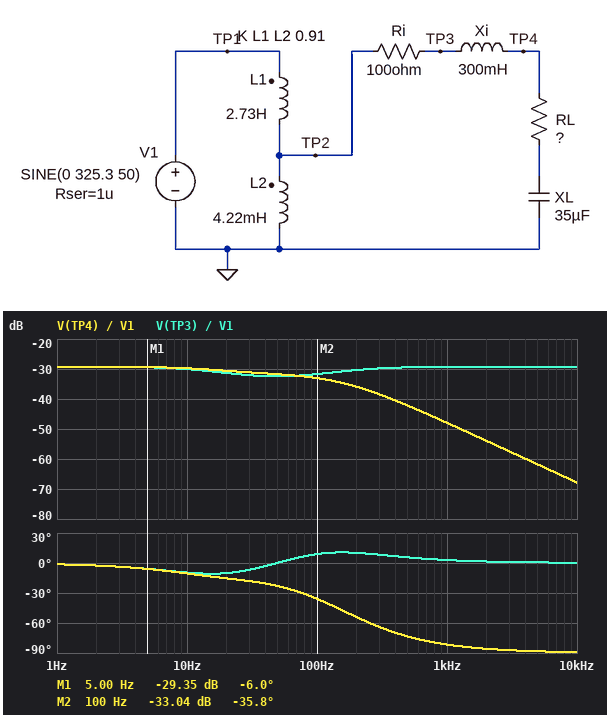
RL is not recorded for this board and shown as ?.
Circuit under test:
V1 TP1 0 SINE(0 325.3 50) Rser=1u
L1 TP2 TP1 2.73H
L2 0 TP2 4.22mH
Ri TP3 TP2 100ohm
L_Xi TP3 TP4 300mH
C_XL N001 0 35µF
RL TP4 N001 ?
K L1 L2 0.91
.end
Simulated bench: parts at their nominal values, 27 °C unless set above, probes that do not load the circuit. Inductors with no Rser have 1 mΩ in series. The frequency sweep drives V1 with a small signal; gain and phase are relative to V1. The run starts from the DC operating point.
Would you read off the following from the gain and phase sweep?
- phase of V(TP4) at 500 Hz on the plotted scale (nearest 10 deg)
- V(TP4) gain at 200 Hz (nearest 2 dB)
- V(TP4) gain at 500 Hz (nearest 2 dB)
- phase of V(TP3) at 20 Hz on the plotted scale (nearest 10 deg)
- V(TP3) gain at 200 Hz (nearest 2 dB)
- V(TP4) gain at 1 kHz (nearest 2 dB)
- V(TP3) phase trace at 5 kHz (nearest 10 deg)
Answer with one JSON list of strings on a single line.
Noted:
["-70 deg", "-36 dB", "-42 dB", "-10 deg", "-30 dB", "-48 dB", "0 deg"]
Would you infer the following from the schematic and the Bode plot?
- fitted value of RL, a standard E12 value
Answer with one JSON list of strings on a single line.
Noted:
["220 Ω"]
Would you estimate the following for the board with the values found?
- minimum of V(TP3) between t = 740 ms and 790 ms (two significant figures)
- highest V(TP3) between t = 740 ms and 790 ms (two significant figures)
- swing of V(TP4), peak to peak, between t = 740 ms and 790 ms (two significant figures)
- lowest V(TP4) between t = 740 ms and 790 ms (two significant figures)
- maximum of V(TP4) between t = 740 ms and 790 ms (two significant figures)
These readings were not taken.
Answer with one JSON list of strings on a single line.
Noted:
["-7.8 V", "7.8 V", "17 V", "-8.4 V", "8.4 V"]
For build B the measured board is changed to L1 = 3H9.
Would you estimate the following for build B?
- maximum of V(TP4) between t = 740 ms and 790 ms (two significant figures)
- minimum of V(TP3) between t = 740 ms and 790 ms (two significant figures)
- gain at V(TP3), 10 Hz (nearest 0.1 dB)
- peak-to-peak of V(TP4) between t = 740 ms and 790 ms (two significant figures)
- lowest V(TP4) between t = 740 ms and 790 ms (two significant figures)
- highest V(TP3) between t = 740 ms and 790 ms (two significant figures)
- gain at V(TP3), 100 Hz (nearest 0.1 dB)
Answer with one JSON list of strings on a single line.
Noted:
["7.1 V", "-6.5 V", "-31.6 dB", "14 V", "-7.1 V", "6.5 V", "-33.2 dB"]
